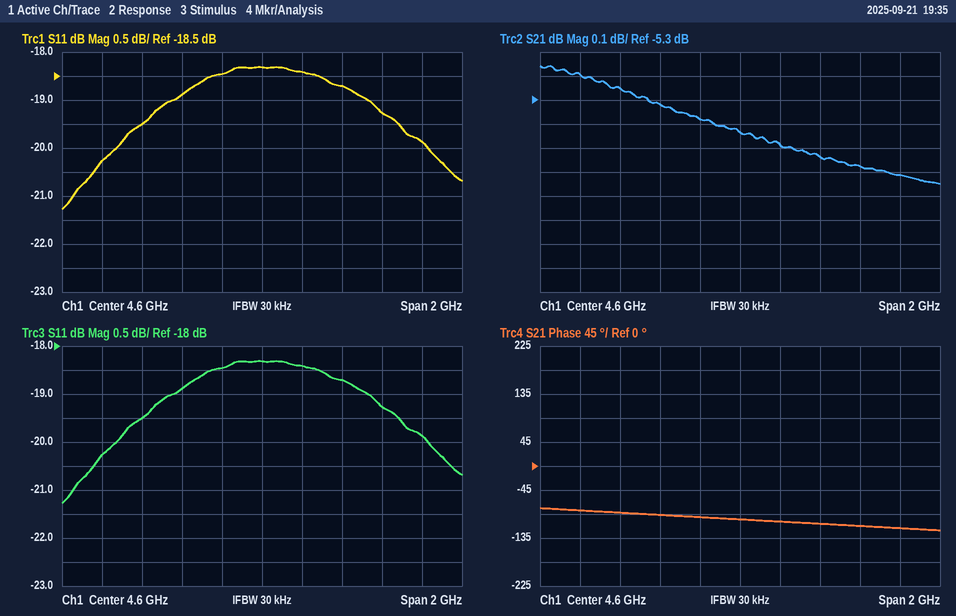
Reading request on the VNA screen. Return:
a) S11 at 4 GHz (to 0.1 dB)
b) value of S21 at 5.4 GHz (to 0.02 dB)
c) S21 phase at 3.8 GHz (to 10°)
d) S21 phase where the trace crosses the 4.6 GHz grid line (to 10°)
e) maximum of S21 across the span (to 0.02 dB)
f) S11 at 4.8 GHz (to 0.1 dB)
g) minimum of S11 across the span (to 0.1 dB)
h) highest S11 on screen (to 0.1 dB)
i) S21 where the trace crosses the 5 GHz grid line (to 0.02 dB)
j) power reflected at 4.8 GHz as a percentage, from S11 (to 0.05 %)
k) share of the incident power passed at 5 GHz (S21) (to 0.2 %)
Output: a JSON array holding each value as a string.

["-19.5 dB", "-5.62 dB", "-80°", "-100°", "-5.16 dB", "-18.4 dB", "-21.3 dB", "-18.3 dB", "-5.54 dB", "1.45 %", "28.0 %"]
